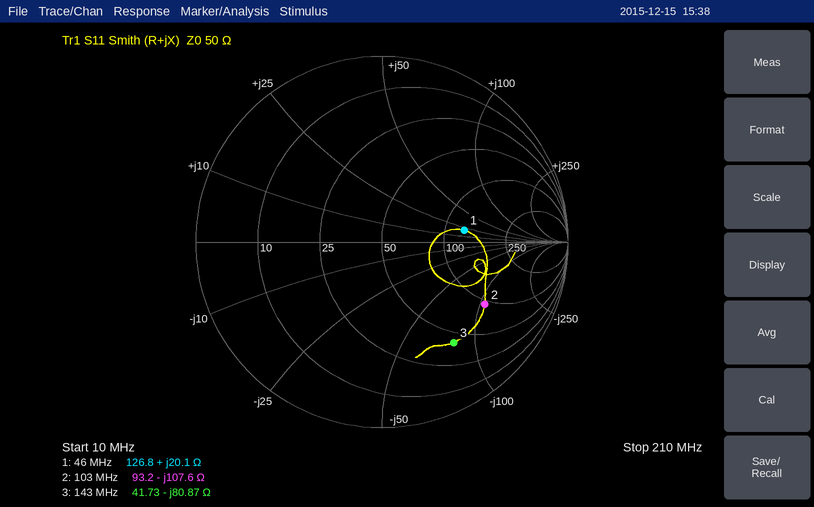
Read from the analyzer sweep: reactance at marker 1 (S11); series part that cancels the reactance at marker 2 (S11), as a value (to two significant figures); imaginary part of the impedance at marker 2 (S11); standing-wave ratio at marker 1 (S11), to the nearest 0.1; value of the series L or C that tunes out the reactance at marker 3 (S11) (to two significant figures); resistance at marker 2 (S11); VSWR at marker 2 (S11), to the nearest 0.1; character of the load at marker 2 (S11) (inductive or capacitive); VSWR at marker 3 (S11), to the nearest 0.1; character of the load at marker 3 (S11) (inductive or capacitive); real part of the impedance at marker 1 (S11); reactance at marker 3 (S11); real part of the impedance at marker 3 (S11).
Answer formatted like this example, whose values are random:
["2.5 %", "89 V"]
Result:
["+20.1 Ω", "170 nH", "-107.6 Ω", "2.6", "90 nH", "93.2 Ω", "4.7", "capacitive", "5.0", "capacitive", "126.8 Ω", "-80.87 Ω", "41.73 Ω"]
